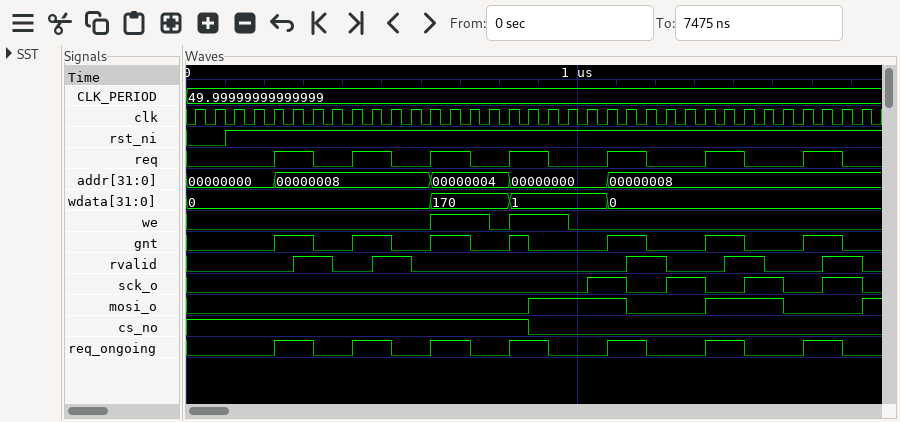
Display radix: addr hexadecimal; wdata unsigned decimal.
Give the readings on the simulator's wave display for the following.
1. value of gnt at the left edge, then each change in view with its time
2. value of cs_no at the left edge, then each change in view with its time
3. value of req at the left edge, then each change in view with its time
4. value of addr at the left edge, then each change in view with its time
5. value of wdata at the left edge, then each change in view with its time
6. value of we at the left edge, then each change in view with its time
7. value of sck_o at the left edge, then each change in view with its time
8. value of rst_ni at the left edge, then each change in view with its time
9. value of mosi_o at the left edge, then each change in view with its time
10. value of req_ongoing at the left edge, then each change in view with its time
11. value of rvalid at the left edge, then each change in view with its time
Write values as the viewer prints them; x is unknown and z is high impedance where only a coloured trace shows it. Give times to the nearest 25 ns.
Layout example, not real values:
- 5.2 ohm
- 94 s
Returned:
- 0, 1 at 225 ns, 0 at 325 ns, 1 at 425 ns, 0 at 525 ns, 1 at 625 ns, 0 at 725 ns, 1 at 825 ns, 0 at 875 ns, 1 at 1075 ns, 0 at 1175 ns, 1 at 1325 ns, 0 at 1425 ns, 1 at 1575 ns, 0 at 1675 ns
- 1, 0 at 875 ns
- 0, 1 at 225 ns, 0 at 325 ns, 1 at 425 ns, 0 at 525 ns, 1 at 625 ns, 0 at 725 ns, 1 at 825 ns, 0 at 925 ns, 1 at 1075 ns, 0 at 1175 ns, 1 at 1325 ns, 0 at 1425 ns, 1 at 1575 ns, 0 at 1675 ns
- 00000000, 00000008 at 225 ns, 00000004 at 625 ns, 00000000 at 825 ns, 00000008 at 1075 ns
- 0, 170 at 625 ns, 1 at 825 ns, 0 at 1075 ns
- 0, 1 at 625 ns, 0 at 775 ns, 1 at 825 ns, 0 at 975 ns
- 0, 1 at 1025 ns, 0 at 1125 ns, 1 at 1225 ns, 0 at 1325 ns, 1 at 1425 ns, 0 at 1525 ns, 1 at 1625 ns, 0 at 1725 ns
- 0, 1 at 100 ns
- 0, 1 at 875 ns, 0 at 1125 ns, 1 at 1325 ns, 0 at 1525 ns, 1 at 1725 ns
- 0, 1 at 225 ns, 0 at 325 ns, 1 at 425 ns, 0 at 525 ns, 1 at 625 ns, 0 at 725 ns, 1 at 825 ns, 0 at 925 ns, 1 at 1075 ns, 0 at 1175 ns, 1 at 1325 ns, 0 at 1425 ns, 1 at 1575 ns, 0 at 1675 ns
- 0, 1 at 275 ns, 0 at 375 ns, 1 at 475 ns, 0 at 575 ns, 1 at 1125 ns, 0 at 1225 ns, 1 at 1375 ns, 0 at 1475 ns, 1 at 1625 ns, 0 at 1725 ns
